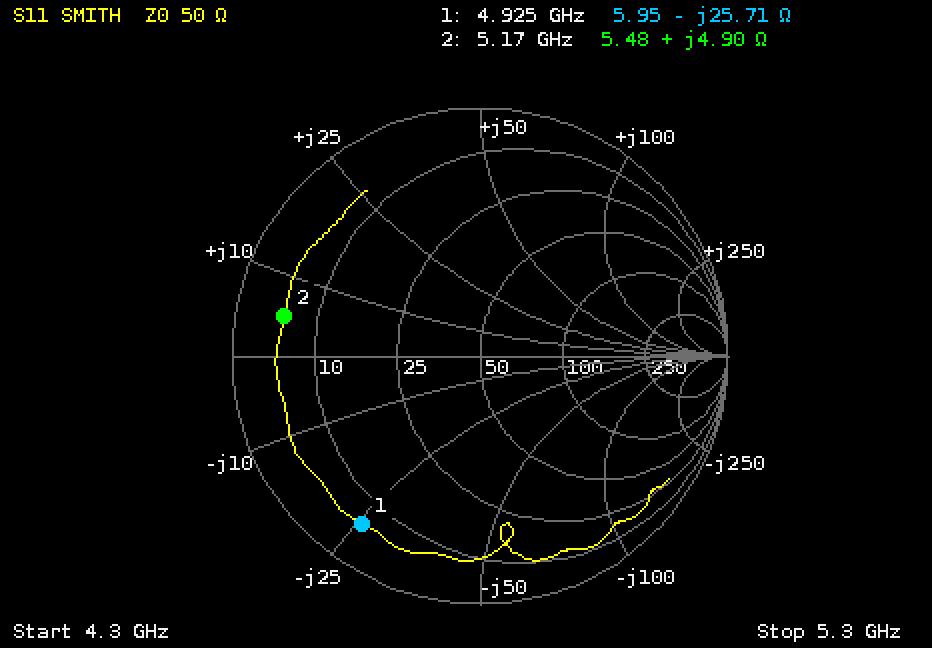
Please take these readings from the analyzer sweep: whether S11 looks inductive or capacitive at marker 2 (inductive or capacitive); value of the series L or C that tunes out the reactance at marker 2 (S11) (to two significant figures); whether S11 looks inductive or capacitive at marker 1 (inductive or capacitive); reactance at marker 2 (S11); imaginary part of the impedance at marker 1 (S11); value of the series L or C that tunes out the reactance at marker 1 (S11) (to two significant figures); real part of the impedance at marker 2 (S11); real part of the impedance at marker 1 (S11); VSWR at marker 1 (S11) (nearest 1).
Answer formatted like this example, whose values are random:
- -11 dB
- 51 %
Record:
- inductive
- 6.3 pF
- capacitive
- +4.90 Ω
- -25.71 Ω
- 830 pH
- 5.48 Ω
- 5.95 Ω
- 11
